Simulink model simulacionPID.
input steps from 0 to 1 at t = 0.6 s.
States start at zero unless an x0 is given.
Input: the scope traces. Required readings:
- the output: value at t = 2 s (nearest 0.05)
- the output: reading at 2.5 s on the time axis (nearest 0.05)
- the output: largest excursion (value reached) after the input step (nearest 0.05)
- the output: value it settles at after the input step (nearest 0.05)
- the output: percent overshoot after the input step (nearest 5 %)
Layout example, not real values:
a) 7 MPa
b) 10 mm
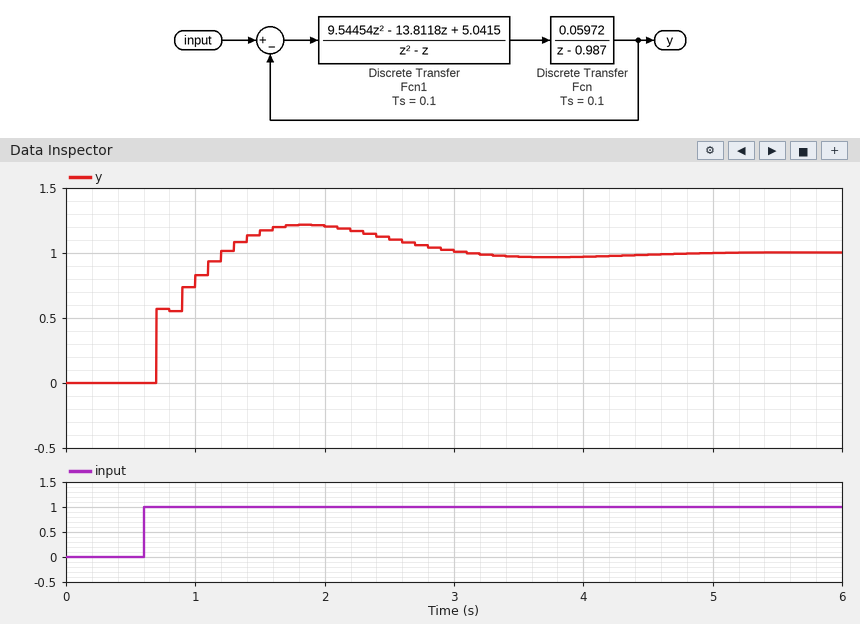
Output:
a) 1.20
b) 1.10
c) 1.20
d) 1.00
e) 20 %
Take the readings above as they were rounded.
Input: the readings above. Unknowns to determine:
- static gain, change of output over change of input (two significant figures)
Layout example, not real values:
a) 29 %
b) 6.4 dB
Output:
a) 1.0
